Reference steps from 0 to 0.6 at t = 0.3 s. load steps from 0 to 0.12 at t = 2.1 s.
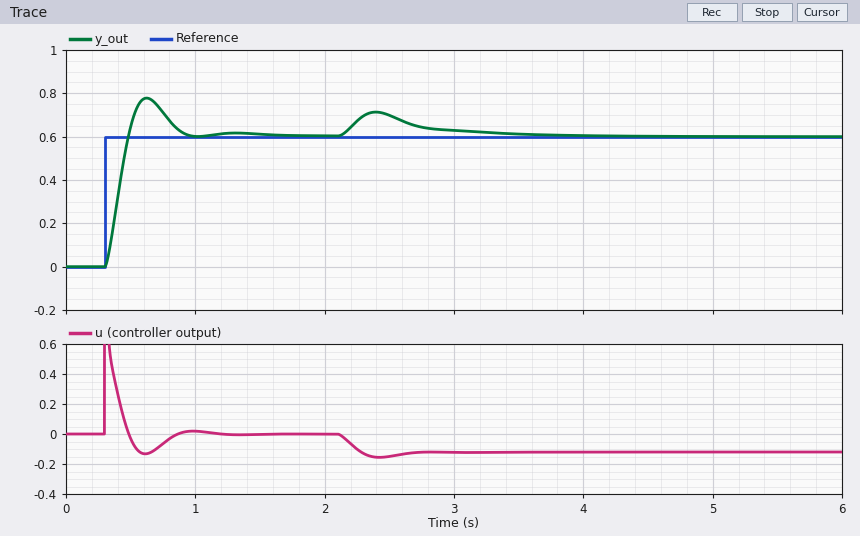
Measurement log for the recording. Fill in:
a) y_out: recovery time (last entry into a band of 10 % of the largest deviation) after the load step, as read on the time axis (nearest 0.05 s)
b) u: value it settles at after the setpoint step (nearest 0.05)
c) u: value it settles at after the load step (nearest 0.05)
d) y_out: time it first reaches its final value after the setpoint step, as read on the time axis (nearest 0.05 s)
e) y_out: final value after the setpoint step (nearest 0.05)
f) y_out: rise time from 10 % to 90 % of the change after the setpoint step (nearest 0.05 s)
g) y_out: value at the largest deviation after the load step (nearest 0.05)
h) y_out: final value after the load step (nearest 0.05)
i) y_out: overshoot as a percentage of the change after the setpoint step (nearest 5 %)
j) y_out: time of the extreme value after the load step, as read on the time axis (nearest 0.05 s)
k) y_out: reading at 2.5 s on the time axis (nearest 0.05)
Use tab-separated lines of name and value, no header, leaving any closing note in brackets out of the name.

y_out: recovery time (last entry into a band of 10 % of the largest deviation) after the load step, as read on the time axis	3.55 s
u: value it settles at after the setpoint step	0.00
u: value it settles at after the load step	-0.10
y_out: time it first reaches its final value after the setpoint step, as read on the time axis	0.50 s
y_out: final value after the setpoint step	0.60
y_out: rise time from 10 % to 90 % of the change after the setpoint step	0.15 s
y_out: value at the largest deviation after the load step	0.70
y_out: final value after the load step	0.60
y_out: overshoot as a percentage of the change after the setpoint step	30 %
y_out: time of the extreme value after the load step, as read on the time axis	2.40 s
y_out: reading at 2.5 s on the time axis	0.70
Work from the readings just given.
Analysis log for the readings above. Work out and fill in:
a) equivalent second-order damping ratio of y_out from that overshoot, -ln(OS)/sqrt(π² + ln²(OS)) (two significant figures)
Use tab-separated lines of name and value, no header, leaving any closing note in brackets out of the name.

equivalent second-order damping ratio of y_out from that overshoot, -ln(OS)/sqrt(π² + ln²(OS))	0.36
